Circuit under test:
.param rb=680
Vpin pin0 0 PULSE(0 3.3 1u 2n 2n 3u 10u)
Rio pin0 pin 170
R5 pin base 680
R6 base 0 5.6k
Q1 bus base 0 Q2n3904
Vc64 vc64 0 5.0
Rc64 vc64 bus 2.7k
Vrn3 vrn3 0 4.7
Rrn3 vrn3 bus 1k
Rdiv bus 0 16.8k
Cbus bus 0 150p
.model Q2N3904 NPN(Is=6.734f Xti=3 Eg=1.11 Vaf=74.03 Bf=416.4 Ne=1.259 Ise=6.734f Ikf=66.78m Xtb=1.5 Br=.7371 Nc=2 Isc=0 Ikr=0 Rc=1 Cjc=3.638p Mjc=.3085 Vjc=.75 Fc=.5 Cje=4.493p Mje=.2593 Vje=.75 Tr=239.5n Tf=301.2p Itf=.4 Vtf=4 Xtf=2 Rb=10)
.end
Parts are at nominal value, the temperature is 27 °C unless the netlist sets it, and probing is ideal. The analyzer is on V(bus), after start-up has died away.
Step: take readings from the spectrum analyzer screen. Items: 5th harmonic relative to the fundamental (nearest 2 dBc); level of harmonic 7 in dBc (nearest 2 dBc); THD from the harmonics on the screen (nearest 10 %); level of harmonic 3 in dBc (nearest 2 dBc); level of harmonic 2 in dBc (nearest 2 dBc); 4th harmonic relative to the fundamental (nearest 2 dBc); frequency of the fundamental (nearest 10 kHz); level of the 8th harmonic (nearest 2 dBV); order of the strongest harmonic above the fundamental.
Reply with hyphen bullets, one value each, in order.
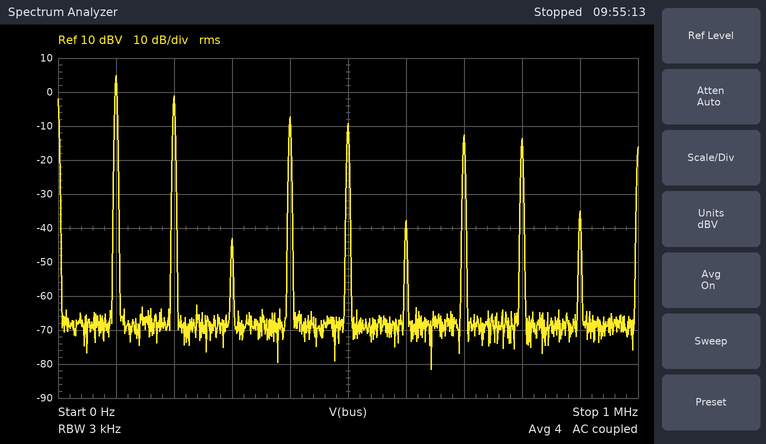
- -14 dBc
- -18 dBc
- 60 %
- -48 dBc
- -6 dBc
- -12 dBc
- 100 kHz
- -14 dBV
- 2
